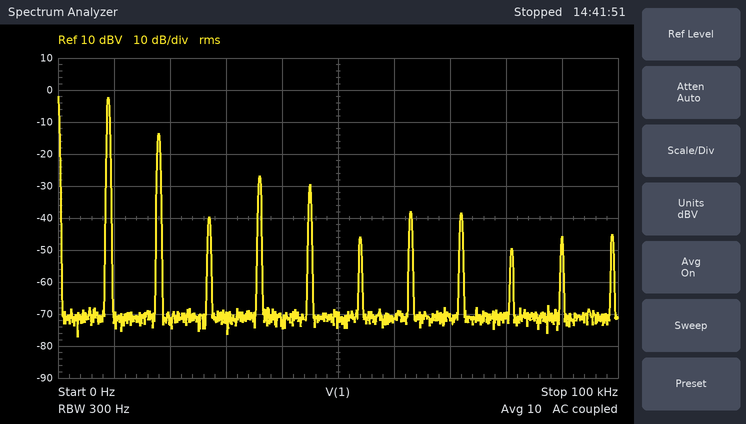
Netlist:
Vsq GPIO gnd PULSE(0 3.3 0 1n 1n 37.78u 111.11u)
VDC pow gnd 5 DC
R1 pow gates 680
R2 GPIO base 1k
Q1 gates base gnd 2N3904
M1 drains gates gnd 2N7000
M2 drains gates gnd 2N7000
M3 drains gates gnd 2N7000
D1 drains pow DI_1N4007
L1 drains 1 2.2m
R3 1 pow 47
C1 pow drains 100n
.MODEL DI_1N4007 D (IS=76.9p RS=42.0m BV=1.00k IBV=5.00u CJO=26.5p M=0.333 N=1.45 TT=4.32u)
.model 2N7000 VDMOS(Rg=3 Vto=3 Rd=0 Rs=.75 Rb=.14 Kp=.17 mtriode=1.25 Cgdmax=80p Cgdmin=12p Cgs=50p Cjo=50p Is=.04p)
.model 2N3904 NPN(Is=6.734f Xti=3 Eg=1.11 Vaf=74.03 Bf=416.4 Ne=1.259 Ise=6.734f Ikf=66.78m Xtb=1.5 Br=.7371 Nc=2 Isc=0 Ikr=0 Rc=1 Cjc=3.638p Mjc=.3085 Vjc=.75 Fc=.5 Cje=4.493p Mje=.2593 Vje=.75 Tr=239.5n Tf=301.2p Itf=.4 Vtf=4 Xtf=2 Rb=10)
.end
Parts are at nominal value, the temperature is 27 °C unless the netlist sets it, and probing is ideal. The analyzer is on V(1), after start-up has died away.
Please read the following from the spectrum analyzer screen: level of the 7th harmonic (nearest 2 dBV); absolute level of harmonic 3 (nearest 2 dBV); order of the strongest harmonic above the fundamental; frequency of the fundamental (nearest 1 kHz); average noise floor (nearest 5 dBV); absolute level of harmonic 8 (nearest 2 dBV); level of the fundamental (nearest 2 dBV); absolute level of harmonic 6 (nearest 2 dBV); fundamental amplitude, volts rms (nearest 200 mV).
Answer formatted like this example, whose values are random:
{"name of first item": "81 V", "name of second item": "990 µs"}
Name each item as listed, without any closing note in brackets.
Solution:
{"level of the 7th harmonic": "-38 dBV", "absolute level of harmonic 3": "-40 dBV", "order of the strongest harmonic above the fundamental": "2", "frequency of the fundamental": "9 kHz", "average noise floor": "-70 dBV", "absolute level of harmonic 8": "-38 dBV", "level of the fundamental": "-2 dBV", "absolute level of harmonic 6": "-46 dBV", "fundamental amplitude, volts rms": "800 mV"}
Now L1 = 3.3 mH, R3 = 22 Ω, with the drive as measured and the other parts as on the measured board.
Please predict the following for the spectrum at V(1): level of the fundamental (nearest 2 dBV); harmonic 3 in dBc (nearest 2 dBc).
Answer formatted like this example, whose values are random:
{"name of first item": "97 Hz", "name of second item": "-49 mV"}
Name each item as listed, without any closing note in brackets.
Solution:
{"level of the fundamental": "-12 dBV", "harmonic 3 in dBc": "-42 dBc"}
